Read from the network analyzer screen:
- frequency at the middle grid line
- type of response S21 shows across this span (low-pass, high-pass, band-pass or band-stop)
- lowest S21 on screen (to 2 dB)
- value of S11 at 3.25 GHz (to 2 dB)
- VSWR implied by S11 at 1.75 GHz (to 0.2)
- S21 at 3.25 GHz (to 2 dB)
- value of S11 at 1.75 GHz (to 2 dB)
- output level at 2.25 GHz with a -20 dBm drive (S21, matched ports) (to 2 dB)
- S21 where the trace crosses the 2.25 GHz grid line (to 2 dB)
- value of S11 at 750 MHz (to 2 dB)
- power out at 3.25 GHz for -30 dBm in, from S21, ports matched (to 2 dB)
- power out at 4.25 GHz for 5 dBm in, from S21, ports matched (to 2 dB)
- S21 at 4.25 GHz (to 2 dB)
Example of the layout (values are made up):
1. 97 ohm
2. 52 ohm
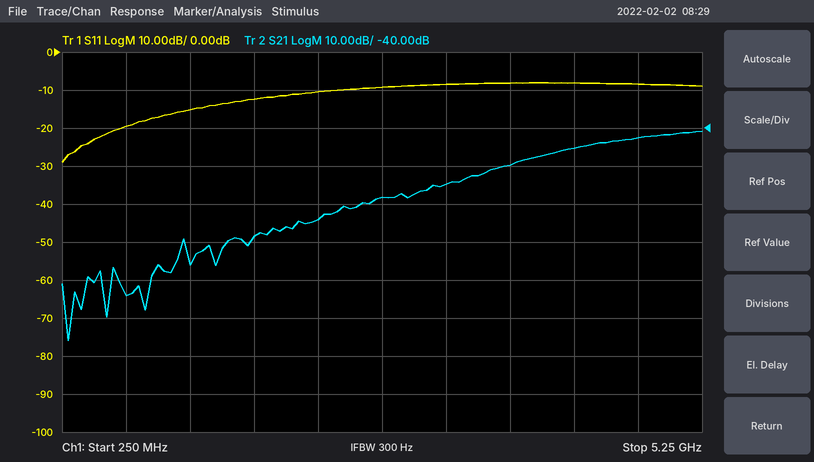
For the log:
1. 2.75 GHz
2. high-pass
3. -96 dB
4. -8 dB
5. 1.6
6. -54 dB
7. -12 dB
8. -84 dBm
9. -64 dB
10. -20 dB
11. -84 dBm
12. -40 dBm
13. -46 dB
